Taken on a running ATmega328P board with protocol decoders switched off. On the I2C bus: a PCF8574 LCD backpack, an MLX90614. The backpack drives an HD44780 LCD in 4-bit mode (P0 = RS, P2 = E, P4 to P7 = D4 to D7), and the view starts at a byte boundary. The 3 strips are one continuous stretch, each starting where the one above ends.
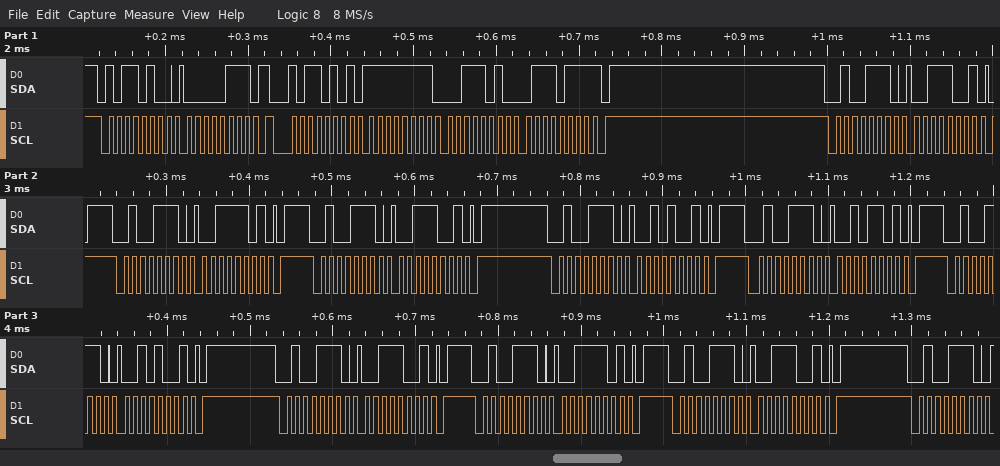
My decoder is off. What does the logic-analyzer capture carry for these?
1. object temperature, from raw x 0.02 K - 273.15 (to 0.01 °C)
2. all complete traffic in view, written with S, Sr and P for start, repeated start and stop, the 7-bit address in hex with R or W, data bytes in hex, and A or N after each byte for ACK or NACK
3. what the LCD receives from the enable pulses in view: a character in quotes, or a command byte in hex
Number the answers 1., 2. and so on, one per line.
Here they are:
1. 28.91 °C
2. S 5AW A 07 A Sr 5AR A FF A 3A A 77 N P S 27W A 39 A P S 27W A 3D A P S 27W A 39 A P S 27W A 29 A P S 27W A 2D A P S 27W A 29 A P S 27W A 39 A P S 27W A 3D A P S 27W A 39 A P S 27W A
3. '2'
